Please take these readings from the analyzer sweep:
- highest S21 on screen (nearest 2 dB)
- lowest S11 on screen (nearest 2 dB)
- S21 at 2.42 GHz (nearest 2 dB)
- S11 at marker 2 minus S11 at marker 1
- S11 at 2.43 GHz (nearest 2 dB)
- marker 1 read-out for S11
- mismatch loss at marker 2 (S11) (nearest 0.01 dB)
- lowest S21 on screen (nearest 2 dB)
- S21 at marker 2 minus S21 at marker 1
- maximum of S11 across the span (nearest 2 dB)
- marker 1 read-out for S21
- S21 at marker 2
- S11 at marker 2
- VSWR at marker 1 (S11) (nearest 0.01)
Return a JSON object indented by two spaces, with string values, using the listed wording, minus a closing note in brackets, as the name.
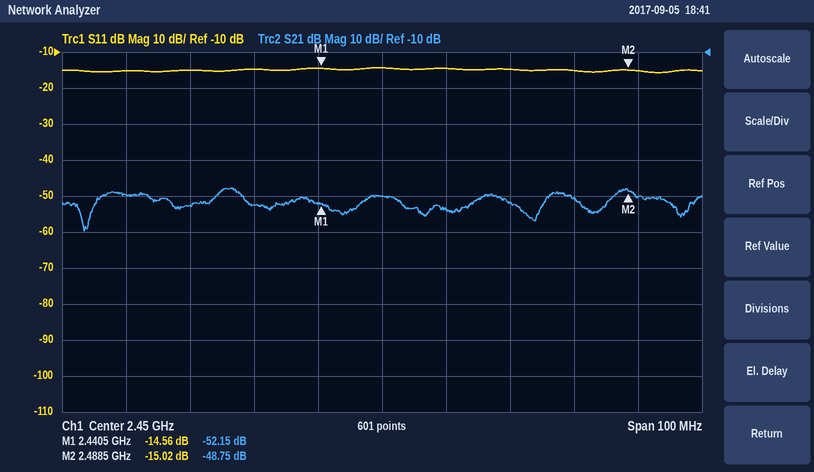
{
  "highest S21 on screen": "-48 dB",
  "lowest S11 on screen": "-16 dB",
  "S21 at 2.42 GHz": "-52 dB",
  "S11 at marker 2 minus S11 at marker 1": "-0.46 dB",
  "S11 at 2.43 GHz": "-14 dB",
  "marker 1 read-out for S11": "-14.56 dB",
  "mismatch loss at marker 2 (S11)": "0.14 dB",
  "lowest S21 on screen": "-60 dB",
  "S21 at marker 2 minus S21 at marker 1": "3.40 dB",
  "maximum of S11 across the span": "-14 dB",
  "marker 1 read-out for S21": "-52.15 dB",
  "S21 at marker 2": "-48.75 dB",
  "S11 at marker 2": "-15.02 dB",
  "VSWR at marker 1 (S11)": "1.46"
}
